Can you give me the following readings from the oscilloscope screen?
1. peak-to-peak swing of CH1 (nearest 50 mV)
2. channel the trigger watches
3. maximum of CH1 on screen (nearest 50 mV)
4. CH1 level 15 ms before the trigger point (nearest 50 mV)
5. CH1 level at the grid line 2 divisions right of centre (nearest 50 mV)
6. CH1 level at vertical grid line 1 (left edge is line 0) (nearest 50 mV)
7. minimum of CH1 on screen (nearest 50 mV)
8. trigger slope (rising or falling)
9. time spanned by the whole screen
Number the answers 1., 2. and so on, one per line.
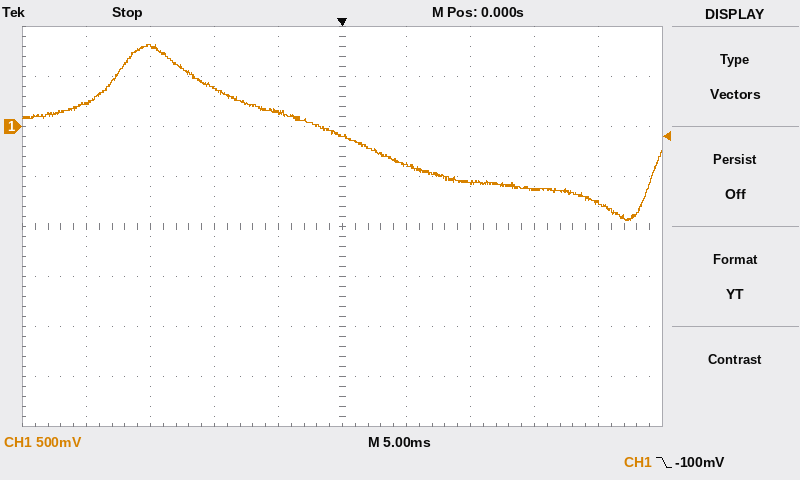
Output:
1. 1.75 V
2. CH1
3. 800 mV
4. 800 mV
5. -550 mV
6. 250 mV
7. -950 mV
8. falling
9. 50 ms
